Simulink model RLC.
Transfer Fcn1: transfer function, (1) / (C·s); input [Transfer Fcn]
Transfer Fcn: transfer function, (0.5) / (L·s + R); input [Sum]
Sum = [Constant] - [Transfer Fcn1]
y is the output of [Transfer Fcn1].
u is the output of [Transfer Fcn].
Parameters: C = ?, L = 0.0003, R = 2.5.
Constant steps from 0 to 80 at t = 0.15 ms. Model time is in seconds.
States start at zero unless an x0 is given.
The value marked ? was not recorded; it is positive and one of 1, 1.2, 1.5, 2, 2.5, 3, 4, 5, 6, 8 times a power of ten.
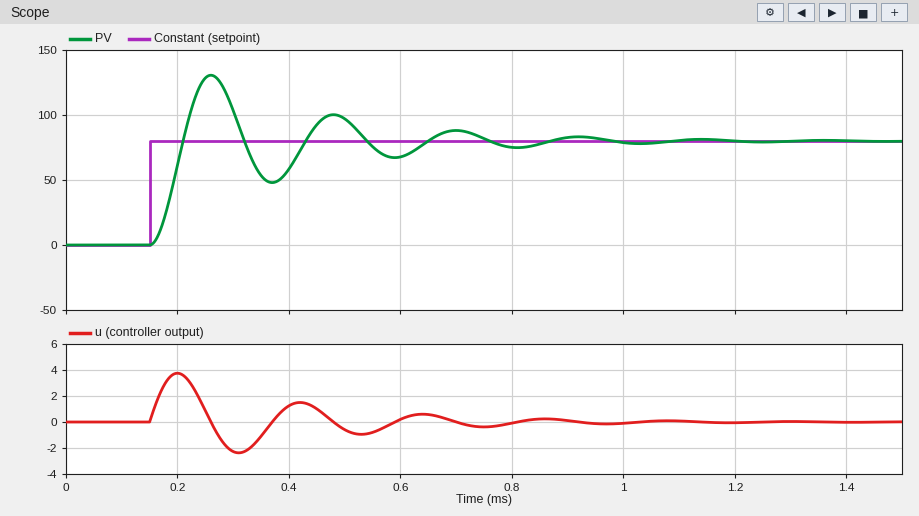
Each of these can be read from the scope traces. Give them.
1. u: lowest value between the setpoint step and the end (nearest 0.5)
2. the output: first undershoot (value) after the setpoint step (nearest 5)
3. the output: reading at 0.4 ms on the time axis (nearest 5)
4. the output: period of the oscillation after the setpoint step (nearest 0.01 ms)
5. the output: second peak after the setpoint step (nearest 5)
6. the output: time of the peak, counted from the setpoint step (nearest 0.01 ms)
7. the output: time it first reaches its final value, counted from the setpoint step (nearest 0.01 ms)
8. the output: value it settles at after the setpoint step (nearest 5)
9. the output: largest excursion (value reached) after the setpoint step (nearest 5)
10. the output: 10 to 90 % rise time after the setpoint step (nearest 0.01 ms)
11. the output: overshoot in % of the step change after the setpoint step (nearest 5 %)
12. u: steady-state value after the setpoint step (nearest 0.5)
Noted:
-2.5
50
60
0.22 ms
100
0.11 ms
0.06 ms
80
130
0.04 ms
65 %
0.0
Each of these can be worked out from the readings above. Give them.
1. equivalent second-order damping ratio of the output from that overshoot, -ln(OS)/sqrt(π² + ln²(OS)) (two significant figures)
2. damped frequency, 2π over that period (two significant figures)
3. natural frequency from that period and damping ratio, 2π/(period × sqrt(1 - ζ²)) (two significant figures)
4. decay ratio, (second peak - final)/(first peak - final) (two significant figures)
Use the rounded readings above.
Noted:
0.14
29 rad/ms
29 rad/ms
0.40
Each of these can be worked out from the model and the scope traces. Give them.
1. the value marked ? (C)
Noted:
2e-06
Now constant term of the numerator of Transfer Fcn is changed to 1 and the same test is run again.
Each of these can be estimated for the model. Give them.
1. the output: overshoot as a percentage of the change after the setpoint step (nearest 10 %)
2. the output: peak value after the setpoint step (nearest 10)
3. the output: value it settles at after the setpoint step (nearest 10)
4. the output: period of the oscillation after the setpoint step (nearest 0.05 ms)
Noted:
70 %
140
80
0.15 ms
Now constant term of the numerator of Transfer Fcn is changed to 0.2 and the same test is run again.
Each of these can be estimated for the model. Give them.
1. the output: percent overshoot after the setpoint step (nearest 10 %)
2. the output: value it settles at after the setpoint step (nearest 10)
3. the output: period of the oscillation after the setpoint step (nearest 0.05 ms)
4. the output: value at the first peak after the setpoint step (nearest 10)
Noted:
50 %
80
0.35 ms
120
